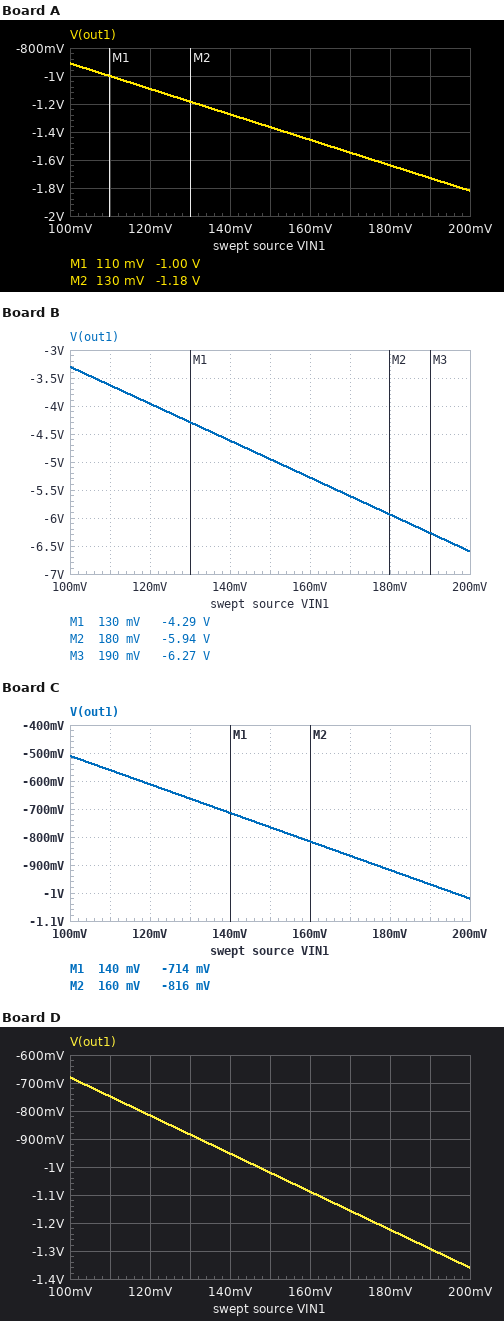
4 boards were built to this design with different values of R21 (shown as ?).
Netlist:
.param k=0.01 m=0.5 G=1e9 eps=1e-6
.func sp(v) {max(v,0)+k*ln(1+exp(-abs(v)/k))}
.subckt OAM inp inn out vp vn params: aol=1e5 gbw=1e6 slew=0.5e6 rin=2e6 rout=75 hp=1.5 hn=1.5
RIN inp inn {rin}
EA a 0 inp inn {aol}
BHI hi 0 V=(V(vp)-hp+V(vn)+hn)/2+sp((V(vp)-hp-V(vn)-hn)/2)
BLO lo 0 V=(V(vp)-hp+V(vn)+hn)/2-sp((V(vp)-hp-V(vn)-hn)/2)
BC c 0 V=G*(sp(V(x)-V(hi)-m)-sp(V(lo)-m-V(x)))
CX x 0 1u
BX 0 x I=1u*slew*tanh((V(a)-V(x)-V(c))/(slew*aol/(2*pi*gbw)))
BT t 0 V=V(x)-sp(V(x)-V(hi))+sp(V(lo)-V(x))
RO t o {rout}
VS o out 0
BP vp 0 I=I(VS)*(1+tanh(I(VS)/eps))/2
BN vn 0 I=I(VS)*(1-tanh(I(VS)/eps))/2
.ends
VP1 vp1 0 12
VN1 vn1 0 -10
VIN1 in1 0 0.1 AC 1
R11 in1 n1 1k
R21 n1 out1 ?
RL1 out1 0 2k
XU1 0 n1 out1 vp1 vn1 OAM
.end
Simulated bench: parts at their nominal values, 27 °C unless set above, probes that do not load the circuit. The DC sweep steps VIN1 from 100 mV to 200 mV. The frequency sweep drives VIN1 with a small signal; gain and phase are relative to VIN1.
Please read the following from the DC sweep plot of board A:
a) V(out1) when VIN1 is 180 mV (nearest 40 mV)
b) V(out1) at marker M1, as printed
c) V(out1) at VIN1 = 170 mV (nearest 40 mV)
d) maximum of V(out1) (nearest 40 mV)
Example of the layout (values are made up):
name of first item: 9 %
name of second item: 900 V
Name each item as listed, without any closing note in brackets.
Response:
V(out1) when VIN1 is 180 mV: -1.64 V
V(out1) at marker M1, as printed: -1.00 V
V(out1) at VIN1 = 170 mV: -1.56 V
maximum of V(out1): -920 mV
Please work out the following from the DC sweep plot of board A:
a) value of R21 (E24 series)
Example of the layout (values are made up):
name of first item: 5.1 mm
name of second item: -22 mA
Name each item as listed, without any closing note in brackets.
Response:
value of R21: 9.1 kΩ
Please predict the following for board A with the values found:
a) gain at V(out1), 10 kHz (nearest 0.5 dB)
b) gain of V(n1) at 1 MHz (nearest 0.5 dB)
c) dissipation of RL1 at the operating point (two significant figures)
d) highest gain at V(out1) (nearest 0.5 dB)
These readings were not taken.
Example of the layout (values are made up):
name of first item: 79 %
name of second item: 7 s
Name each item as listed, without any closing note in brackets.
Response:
gain at V(out1), 10 kHz: 19.0 dB
gain of V(n1) at 1 MHz: -1.0 dB
dissipation of RL1 at the operating point: 410 µW
highest gain at V(out1): 19.0 dB
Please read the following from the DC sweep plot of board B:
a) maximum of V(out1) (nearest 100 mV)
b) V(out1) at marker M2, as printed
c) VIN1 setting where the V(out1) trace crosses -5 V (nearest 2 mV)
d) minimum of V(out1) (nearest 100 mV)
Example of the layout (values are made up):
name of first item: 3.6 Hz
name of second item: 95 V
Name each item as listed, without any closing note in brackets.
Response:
maximum of V(out1): -3.3 V
V(out1) at marker M2, as printed: -5.94 V
VIN1 setting where the V(out1) trace crosses -5 V: 152 mV
minimum of V(out1): -6.6 V
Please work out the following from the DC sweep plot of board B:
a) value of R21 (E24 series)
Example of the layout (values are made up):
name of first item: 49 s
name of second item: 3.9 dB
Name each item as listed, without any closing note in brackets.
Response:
value of R21: 33 kΩ
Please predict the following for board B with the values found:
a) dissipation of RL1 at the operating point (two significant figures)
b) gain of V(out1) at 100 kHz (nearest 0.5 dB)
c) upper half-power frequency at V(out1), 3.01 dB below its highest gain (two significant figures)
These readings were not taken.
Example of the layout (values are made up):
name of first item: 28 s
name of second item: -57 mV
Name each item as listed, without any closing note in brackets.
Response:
dissipation of RL1 at the operating point: 5.4 mW
gain of V(out1) at 100 kHz: 19.0 dB
upper half-power frequency at V(out1), 3.01 dB below its highest gain: 28 kHz
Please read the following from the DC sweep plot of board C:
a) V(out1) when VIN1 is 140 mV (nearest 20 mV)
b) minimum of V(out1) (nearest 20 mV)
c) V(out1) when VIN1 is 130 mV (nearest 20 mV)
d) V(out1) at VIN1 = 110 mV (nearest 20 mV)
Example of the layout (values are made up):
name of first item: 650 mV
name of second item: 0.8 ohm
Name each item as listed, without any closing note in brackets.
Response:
V(out1) when VIN1 is 140 mV: -720 mV
minimum of V(out1): -1.02 V
V(out1) when VIN1 is 130 mV: -660 mV
V(out1) at VIN1 = 110 mV: -560 mV
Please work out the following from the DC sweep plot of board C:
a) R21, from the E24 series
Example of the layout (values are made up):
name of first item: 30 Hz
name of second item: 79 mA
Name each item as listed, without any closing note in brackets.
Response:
R21, from the E24 series: 5.1 kΩ
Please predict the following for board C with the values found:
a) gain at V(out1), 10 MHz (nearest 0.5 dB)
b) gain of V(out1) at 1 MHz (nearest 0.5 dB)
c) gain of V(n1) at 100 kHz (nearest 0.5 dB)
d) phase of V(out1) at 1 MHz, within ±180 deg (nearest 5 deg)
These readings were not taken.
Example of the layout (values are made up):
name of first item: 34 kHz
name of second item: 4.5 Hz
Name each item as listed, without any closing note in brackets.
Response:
gain at V(out1), 10 MHz: -22.0 dB
gain of V(out1) at 1 MHz: -2.0 dB
gain of V(n1) at 100 kHz: -7.0 dB
phase of V(out1) at 1 MHz, within ±180 deg: 100 deg
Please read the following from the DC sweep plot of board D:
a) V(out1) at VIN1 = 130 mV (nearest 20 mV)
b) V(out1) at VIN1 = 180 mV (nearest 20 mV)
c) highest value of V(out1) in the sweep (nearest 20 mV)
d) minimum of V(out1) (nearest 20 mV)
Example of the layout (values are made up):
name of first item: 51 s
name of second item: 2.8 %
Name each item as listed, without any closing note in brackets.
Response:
V(out1) at VIN1 = 130 mV: -880 mV
V(out1) at VIN1 = 180 mV: -1.22 V
highest value of V(out1) in the sweep: -680 mV
minimum of V(out1): -1.36 V
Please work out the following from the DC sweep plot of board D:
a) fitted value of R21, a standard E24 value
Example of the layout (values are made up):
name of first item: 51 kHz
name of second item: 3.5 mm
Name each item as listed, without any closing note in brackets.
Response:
fitted value of R21, a standard E24 value: 6.8 kΩ
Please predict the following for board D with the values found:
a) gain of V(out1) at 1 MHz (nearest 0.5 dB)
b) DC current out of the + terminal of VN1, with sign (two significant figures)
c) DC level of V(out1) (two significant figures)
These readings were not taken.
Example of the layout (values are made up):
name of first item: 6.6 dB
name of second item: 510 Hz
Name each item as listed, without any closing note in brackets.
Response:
gain of V(out1) at 1 MHz: -1.5 dB
DC current out of the + terminal of VN1, with sign: -440 µA
DC level of V(out1): -680 mV
